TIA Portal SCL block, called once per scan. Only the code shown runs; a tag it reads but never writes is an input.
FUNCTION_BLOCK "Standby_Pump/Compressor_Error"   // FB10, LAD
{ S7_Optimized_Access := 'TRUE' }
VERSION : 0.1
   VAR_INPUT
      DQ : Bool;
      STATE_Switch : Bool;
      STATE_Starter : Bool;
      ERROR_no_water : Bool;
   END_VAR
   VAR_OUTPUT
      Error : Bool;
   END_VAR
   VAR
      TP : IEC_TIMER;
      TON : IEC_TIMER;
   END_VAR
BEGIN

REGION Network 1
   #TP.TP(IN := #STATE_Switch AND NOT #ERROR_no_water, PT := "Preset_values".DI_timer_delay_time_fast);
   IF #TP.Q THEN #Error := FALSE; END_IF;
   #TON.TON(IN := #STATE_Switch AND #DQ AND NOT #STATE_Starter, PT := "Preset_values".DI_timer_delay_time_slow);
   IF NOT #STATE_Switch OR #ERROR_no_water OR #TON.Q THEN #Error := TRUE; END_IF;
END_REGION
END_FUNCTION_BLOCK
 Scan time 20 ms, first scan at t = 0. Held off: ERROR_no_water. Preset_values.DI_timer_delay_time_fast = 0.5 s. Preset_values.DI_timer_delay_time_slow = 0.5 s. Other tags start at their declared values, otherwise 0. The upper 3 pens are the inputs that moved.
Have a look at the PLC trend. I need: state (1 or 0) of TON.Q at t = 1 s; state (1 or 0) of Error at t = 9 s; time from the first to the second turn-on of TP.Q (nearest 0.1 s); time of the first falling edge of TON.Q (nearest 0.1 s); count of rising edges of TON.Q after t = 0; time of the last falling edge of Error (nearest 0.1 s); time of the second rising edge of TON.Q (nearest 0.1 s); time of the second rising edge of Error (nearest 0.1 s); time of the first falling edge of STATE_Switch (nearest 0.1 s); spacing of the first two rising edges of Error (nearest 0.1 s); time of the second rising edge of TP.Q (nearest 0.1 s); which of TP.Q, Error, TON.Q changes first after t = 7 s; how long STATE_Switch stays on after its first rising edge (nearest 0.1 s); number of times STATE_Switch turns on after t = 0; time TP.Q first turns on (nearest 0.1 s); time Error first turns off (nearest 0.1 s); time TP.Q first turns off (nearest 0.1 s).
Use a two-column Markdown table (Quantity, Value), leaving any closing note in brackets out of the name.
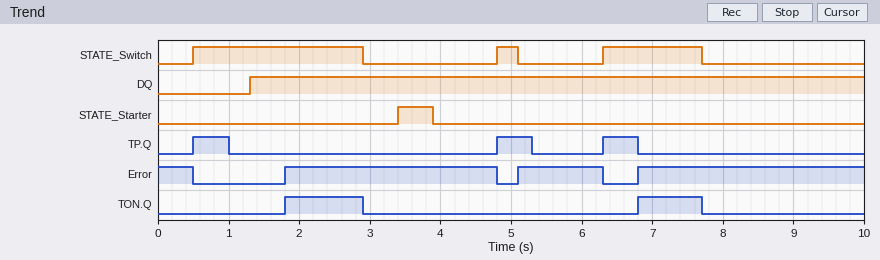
| Quantity | Value |
|---|---|
| state (1 or 0) of TON.Q at t = 1 s | 0 |
| state (1 or 0) of Error at t = 9 s | 1 |
| time from the first to the second turn-on of TP.Q | 4.3 s |
| time of the first falling edge of TON.Q | 2.9 s |
| count of rising edges of TON.Q after t = 0 | 2 |
| time of the last falling edge of Error | 6.3 s |
| time of the second rising edge of TON.Q | 6.8 s |
| time of the second rising edge of Error | 5.1 s |
| time of the first falling edge of STATE_Switch | 2.9 s |
| spacing of the first two rising edges of Error | 3.3 s |
| time of the second rising edge of TP.Q | 4.8 s |
| which of TP.Q, Error, TON.Q changes first after t = 7 s | TON.Q |
| how long STATE_Switch stays on after its first rising edge | 2.4 s |
| number of times STATE_Switch turns on after t = 0 | 3 |
| time TP.Q first turns on | 0.5 s |
| time Error first turns off | 0.5 s |
| time TP.Q first turns off | 1.0 s |
